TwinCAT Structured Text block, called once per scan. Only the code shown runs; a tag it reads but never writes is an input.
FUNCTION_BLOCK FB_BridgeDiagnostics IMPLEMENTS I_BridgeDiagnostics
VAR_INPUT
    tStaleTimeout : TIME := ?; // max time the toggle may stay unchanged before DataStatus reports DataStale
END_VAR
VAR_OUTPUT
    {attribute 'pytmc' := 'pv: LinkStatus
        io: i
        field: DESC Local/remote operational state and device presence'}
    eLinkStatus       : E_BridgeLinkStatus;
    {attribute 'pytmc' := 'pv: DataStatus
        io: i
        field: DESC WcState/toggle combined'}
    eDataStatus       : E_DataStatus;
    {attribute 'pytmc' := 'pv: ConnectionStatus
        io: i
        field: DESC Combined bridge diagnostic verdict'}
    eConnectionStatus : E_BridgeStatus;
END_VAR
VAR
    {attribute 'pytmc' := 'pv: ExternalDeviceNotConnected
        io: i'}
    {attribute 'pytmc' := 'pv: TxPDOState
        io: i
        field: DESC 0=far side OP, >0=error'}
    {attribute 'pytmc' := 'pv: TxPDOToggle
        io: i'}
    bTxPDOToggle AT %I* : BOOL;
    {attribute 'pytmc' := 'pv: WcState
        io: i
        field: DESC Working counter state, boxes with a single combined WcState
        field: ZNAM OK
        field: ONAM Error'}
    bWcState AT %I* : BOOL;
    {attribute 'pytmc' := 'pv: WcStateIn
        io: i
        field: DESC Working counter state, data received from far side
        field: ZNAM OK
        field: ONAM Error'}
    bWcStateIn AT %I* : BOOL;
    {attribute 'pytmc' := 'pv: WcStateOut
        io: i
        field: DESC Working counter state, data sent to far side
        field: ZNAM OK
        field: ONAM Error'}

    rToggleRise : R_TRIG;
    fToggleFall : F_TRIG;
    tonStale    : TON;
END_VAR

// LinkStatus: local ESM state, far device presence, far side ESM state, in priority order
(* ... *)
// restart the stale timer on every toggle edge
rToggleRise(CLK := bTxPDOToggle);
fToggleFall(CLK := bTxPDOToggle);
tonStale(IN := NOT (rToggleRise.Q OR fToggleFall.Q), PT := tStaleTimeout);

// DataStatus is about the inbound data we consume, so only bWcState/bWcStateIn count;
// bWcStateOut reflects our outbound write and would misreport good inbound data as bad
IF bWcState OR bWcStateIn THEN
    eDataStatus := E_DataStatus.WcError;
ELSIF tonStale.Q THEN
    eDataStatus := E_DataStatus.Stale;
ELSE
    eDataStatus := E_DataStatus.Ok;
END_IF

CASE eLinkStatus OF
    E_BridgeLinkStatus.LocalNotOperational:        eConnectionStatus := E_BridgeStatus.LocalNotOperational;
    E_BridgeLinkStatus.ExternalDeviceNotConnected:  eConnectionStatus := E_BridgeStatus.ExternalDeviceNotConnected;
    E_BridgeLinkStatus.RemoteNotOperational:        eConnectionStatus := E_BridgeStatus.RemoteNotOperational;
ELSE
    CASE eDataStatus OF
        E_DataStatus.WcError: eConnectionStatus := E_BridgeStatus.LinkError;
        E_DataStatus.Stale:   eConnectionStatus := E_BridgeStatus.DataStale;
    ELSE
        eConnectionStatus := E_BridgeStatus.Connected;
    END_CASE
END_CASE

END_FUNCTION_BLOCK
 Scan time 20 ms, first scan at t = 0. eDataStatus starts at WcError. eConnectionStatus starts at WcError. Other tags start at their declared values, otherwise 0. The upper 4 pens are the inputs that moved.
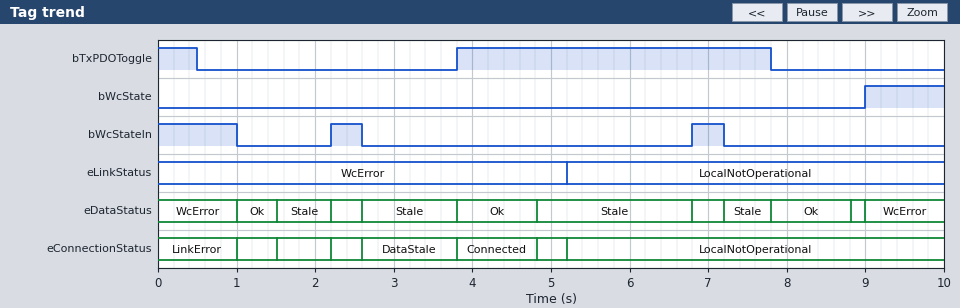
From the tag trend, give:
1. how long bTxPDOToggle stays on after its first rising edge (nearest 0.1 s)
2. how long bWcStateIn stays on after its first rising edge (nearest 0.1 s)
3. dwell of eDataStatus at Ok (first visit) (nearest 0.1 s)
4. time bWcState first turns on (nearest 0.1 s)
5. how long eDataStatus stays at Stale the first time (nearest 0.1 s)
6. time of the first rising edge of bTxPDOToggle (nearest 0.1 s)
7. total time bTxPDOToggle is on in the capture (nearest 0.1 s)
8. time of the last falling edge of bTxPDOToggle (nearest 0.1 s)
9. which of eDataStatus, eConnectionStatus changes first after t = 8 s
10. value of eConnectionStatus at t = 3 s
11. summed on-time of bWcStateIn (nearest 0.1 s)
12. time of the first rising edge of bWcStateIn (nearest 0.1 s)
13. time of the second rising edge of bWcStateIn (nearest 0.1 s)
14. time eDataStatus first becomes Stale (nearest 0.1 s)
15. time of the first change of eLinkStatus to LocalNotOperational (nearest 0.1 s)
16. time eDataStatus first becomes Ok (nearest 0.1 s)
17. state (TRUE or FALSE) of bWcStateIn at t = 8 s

4.0 s
0.4 s
0.5 s
9.0 s
0.7 s
3.8 s
4.5 s
7.8 s
eDataStatus
DataStale
1.8 s
2.2 s
6.8 s
1.5 s
5.2 s
1.0 s
FALSE
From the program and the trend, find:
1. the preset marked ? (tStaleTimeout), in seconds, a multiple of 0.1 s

1.0 s
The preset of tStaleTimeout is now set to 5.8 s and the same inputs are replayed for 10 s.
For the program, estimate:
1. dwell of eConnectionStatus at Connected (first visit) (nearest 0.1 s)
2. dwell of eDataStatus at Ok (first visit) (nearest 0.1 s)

1.2 s
1.2 s
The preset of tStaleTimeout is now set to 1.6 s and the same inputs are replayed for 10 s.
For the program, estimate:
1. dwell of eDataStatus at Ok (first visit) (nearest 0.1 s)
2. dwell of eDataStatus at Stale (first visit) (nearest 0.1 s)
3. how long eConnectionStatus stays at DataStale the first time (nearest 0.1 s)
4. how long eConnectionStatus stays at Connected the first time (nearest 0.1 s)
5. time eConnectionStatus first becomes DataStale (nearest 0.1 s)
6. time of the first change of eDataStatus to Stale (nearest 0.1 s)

1.1 s
0.1 s
0.1 s
1.1 s
2.1 s
2.1 s
